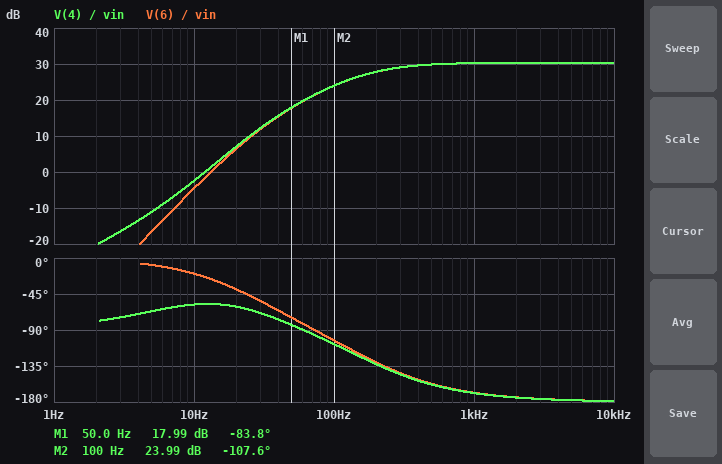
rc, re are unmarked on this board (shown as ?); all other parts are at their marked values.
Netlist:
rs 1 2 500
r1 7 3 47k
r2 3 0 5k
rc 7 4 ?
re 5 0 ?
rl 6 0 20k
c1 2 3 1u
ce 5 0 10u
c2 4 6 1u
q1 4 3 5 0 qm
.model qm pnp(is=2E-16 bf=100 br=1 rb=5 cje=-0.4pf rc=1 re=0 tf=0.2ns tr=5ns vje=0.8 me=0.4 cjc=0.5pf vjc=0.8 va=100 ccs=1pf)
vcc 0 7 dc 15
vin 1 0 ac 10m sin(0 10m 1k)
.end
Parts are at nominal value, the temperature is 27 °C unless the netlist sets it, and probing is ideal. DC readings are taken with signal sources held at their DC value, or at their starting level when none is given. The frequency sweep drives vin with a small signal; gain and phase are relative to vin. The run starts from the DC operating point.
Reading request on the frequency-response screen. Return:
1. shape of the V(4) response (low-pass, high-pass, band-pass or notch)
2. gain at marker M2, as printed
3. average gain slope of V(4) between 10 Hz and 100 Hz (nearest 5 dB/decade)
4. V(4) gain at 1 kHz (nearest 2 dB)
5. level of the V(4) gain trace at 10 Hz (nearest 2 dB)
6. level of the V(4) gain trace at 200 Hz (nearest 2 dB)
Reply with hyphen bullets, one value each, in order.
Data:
- high-pass
- 23.99 dB
- 25 dB/decade
- 30 dB
- -2 dB
- 28 dB
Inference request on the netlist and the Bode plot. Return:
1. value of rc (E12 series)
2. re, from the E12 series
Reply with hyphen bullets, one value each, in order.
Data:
- 4.7 kΩ
- 2.7 kΩ
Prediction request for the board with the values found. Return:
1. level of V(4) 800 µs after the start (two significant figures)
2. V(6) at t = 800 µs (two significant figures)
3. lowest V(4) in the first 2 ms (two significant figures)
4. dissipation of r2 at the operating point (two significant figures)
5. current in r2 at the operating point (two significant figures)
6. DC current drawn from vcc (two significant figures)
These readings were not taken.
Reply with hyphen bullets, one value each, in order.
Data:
- -13 V
- 340 mV
- -14 V
- 410 µW
- 290 µA
- 550 µA
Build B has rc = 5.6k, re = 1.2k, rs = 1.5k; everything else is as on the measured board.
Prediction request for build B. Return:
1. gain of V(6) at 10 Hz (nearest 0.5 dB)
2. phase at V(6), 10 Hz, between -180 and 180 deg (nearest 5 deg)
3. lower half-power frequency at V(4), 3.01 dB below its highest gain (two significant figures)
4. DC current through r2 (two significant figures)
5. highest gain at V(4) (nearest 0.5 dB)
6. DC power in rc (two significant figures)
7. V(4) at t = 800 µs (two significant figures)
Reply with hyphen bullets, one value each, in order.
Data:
- -0.5 dB
- -45 deg
- 310 Hz
- 280 µA
- 35.0 dB
- 1.8 mW
- -11 V
